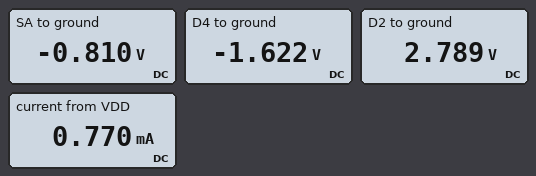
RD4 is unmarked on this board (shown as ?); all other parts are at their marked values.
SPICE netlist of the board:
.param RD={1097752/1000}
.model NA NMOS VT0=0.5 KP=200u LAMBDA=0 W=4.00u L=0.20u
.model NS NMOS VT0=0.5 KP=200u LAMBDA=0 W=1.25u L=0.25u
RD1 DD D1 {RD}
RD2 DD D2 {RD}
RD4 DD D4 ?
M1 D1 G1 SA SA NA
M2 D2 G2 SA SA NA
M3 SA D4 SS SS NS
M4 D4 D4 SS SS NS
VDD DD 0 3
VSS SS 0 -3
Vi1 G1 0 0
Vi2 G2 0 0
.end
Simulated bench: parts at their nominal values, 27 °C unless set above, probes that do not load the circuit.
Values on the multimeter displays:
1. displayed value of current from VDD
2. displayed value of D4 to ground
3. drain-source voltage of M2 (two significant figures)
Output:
0.770 mA
-1.622 V
3.6 V
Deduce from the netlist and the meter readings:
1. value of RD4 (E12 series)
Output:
12 kΩ
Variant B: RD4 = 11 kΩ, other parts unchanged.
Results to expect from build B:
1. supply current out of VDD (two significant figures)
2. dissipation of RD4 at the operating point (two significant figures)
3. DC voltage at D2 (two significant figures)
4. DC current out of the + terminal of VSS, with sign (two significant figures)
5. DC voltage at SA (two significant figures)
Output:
830 µA
1.9 mW
2.8 V
-830 µA
-820 mV
